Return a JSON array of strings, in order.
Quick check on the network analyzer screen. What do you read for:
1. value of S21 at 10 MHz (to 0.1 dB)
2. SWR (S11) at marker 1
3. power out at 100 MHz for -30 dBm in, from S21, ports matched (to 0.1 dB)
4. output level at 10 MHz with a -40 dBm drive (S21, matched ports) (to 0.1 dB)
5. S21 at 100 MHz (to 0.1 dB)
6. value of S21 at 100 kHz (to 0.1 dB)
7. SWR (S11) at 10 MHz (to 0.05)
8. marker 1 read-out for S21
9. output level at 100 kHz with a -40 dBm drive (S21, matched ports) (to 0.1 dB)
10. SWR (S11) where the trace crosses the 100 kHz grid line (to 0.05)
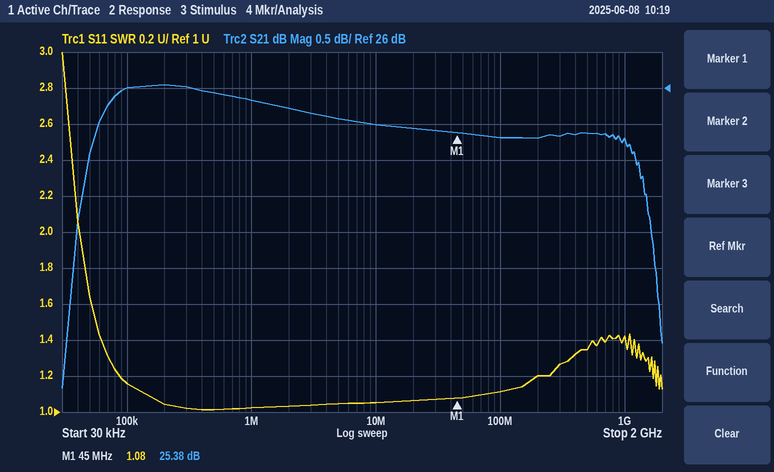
["25.5 dB", "1.08", "-4.7 dBm", "-14.5 dBm", "25.3 dB", "26.0 dB", "1.05", "25.38 dB", "-14.0 dBm", "1.15"]
